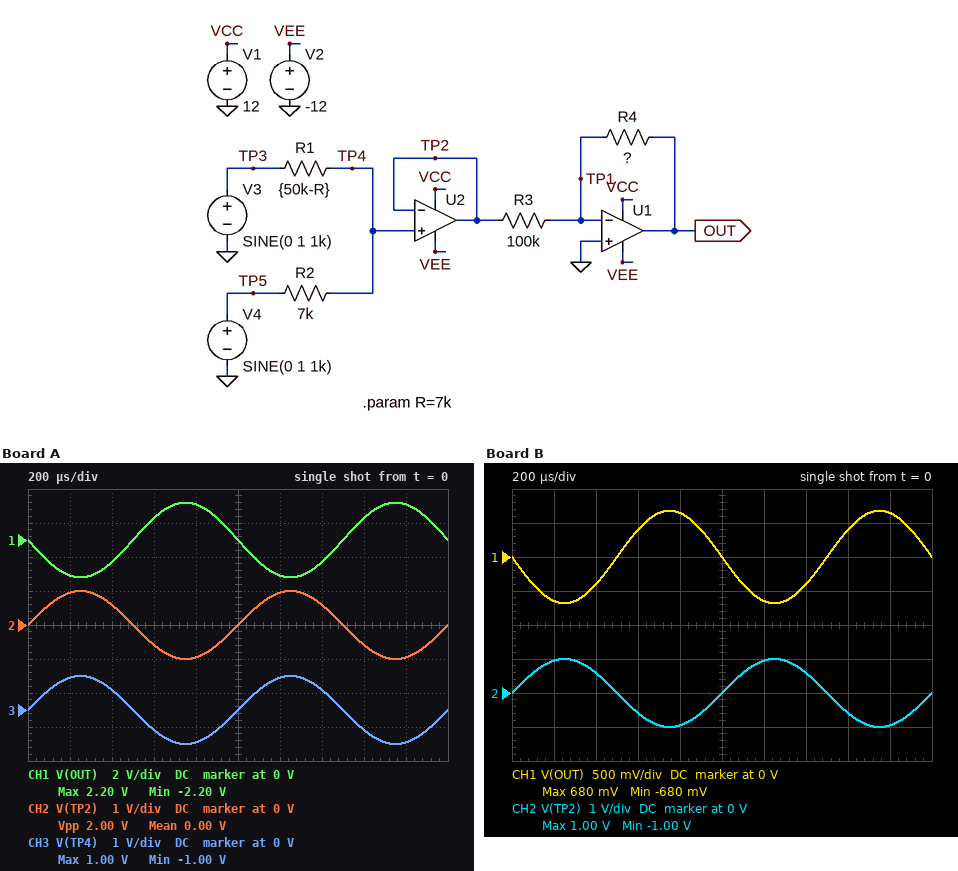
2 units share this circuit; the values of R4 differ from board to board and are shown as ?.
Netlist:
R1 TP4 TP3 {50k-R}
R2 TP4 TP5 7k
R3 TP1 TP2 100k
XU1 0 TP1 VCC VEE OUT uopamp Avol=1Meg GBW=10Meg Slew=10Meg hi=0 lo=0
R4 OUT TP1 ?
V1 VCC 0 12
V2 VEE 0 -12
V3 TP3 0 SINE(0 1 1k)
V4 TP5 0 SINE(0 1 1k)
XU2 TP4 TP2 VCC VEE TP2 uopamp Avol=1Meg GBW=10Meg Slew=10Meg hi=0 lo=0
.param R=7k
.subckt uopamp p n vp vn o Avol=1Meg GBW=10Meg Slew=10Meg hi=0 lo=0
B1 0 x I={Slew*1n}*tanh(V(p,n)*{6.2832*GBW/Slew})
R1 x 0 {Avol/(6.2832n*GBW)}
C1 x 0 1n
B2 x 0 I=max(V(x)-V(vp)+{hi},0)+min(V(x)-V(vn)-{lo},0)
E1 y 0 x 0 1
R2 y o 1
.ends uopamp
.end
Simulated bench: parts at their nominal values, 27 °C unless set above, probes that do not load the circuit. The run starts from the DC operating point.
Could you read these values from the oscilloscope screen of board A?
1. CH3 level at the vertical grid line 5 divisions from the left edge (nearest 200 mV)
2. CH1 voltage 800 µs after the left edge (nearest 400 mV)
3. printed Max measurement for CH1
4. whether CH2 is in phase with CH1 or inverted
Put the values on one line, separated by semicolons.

0 V; 2.0 V; 2.20 V; inverted
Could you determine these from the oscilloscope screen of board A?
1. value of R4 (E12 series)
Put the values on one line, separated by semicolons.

220 kΩ
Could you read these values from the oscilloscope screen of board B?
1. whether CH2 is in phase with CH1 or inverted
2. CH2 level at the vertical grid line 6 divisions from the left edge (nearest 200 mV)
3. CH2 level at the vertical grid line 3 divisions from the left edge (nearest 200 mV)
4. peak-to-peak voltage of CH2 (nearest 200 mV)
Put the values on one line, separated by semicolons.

inverted; 1.0 V; -600 mV; 2.0 V
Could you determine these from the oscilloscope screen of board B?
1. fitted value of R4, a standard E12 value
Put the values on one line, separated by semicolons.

68 kΩ
